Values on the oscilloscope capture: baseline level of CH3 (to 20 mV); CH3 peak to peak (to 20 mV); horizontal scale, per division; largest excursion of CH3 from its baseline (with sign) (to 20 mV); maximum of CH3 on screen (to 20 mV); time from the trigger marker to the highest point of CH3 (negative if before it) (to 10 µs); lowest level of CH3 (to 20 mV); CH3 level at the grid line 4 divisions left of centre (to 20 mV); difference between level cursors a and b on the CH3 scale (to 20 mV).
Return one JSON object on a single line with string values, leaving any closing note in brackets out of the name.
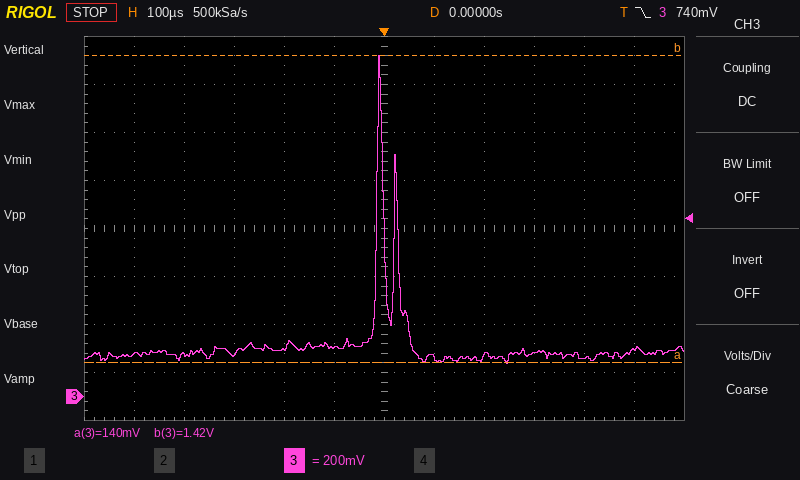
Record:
{"baseline level of CH3": "180 mV", "CH3 peak to peak": "1.28 V", "horizontal scale, per division": "100 µs", "largest excursion of CH3 from its baseline (with sign)": "+1.24 V", "maximum of CH3 on screen": "1.42 V", "time from the trigger marker to the highest point of CH3 (negative if before it)": "-10 µs", "lowest level of CH3": "140 mV", "CH3 level at the grid line 4 divisions left of centre": "180 mV", "difference between level cursors a and b on the CH3 scale": "1.28 V"}
